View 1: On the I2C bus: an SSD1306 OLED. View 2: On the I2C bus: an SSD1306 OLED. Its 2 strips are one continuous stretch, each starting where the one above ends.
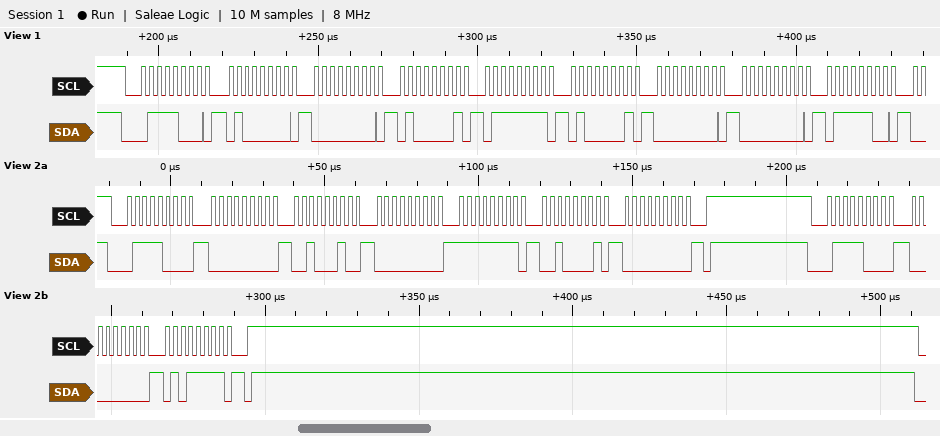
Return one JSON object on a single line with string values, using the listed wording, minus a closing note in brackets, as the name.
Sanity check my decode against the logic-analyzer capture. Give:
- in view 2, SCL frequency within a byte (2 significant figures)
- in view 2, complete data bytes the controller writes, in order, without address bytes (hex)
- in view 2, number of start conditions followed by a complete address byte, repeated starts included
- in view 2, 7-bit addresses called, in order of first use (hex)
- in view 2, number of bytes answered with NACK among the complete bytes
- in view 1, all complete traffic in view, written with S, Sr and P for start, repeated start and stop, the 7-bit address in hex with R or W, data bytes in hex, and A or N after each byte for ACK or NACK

{"in view 2, SCL frequency within a byte": "400 kHz", "in view 2, complete data bytes the controller writes, in order, without address bytes": "00 22 00 FF 21 00 00 5F", "in view 2, number of start conditions followed by a complete address byte, repeated starts included": "2", "in view 2, 7-bit addresses called, in order of first use": "0x3C", "in view 2, number of bytes answered with NACK among the complete bytes": "0", "in view 1, all complete traffic in view, written with S, Sr and P for start, repeated start and stop, the 7-bit address in hex with R or W, data bytes in hex, and A or N after each byte for ACK or NACK": "S 3CW A 40 A 00 A 41 A 7F A 41 A 00 A 00 A 7C A"}
